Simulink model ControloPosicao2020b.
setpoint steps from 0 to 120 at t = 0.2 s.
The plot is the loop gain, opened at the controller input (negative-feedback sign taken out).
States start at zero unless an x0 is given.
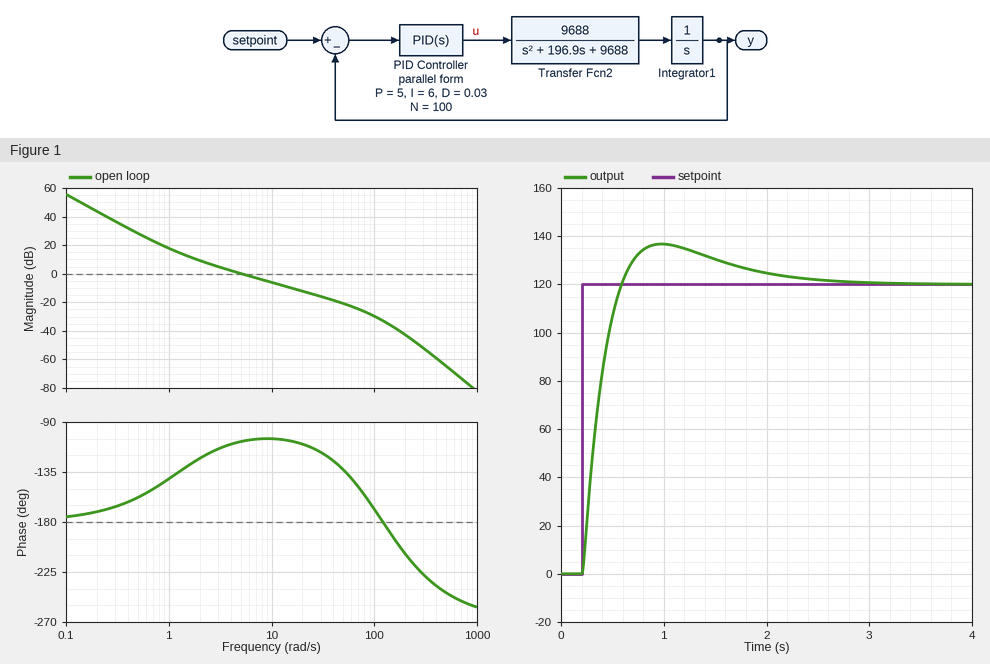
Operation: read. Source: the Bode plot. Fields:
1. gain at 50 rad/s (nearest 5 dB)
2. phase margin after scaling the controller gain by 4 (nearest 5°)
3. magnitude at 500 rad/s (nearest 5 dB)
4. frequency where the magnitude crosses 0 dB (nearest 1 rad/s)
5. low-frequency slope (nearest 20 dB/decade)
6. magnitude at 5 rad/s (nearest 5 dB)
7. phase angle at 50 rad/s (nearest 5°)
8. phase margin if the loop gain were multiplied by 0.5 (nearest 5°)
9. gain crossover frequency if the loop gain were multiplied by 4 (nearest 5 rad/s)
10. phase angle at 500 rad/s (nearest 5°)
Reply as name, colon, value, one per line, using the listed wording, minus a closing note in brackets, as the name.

gain at 50 rad/s: -20 dB
phase margin after scaling the controller gain by 4: 70°
magnitude at 500 rad/s: -65 dB
frequency where the magnitude crosses 0 dB: 5 rad/s
low-frequency slope: -40 dB/decade
magnitude at 5 rad/s: 0 dB
phase angle at 50 rad/s: -135°
phase margin if the loop gain were multiplied by 0.5: 65°
gain crossover frequency if the loop gain were multiplied by 4: 20 rad/s
phase angle at 500 rad/s: -245°
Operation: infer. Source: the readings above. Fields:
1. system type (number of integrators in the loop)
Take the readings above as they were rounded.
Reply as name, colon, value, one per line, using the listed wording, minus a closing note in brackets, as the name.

system type: 2
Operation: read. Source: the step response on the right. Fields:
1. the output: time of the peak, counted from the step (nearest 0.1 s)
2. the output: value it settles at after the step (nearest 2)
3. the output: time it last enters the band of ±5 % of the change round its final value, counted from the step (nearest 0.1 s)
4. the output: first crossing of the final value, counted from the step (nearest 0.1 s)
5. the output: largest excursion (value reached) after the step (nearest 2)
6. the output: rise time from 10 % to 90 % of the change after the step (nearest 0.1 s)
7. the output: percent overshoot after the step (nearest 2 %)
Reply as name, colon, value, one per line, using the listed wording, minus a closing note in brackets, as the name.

the output: time of the peak, counted from the step: 0.8 s
the output: value it settles at after the step: 120
the output: time it last enters the band of ±5 % of the change round its final value, counted from the step: 1.7 s
the output: first crossing of the final value, counted from the step: 0.4 s
the output: largest excursion (value reached) after the step: 136
the output: rise time from 10 % to 90 % of the change after the step: 0.3 s
the output: percent overshoot after the step: 14 %
